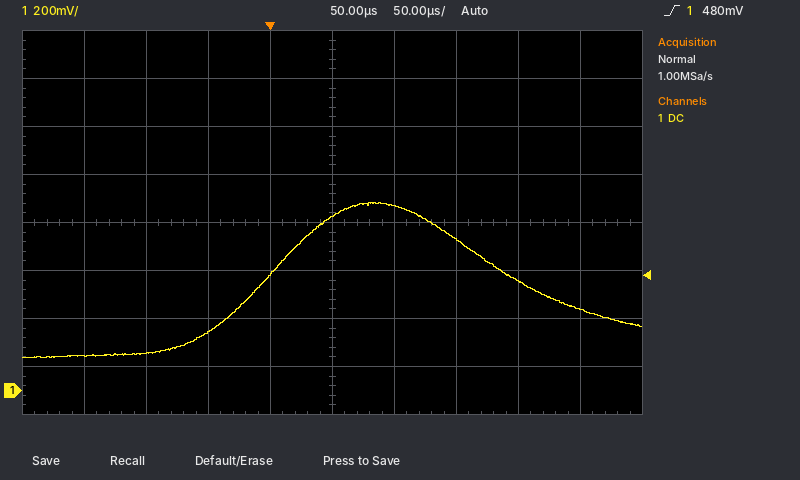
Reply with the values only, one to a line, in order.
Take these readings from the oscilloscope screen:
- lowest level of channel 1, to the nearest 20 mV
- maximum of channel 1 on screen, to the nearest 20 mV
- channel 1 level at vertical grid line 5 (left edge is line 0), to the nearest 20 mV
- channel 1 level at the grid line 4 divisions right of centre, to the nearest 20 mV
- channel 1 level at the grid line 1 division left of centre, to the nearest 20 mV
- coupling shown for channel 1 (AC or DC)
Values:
140 mV
780 mV
720 mV
340 mV
480 mV
DC
